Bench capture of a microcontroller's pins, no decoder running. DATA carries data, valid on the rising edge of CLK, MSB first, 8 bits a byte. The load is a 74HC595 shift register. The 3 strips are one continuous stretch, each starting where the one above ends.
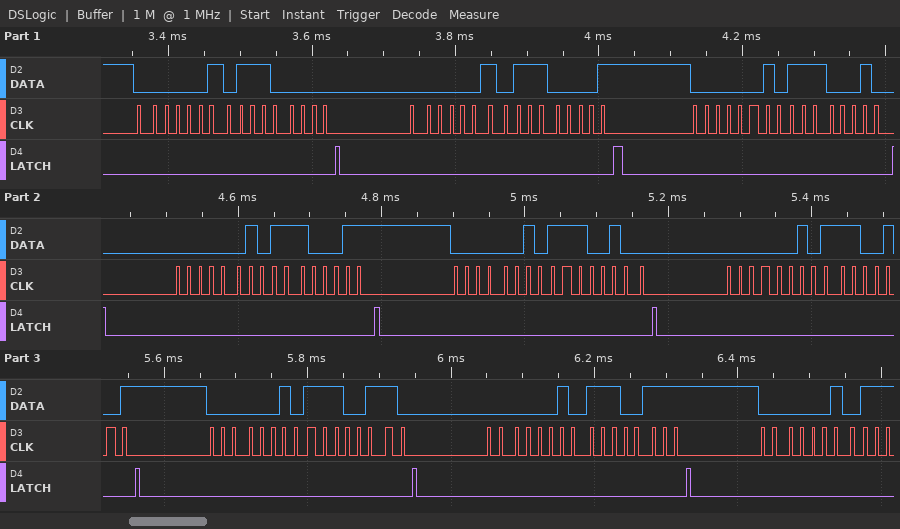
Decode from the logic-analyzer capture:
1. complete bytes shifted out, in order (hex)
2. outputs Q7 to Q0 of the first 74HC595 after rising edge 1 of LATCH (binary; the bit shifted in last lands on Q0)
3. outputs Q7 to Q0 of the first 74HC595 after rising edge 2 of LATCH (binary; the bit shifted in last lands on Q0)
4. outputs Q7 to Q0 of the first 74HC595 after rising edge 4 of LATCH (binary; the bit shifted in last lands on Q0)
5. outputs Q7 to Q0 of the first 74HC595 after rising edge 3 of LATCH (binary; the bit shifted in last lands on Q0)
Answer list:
0x02 0xE0 0x02 0xE1 0x02 0xE2 0x02 0xE3 0x02 0xE4 0x02 0xE5 0x02 0xE6 0x02 0xE7 0x02
11100000
11100001
11100011
11100010
